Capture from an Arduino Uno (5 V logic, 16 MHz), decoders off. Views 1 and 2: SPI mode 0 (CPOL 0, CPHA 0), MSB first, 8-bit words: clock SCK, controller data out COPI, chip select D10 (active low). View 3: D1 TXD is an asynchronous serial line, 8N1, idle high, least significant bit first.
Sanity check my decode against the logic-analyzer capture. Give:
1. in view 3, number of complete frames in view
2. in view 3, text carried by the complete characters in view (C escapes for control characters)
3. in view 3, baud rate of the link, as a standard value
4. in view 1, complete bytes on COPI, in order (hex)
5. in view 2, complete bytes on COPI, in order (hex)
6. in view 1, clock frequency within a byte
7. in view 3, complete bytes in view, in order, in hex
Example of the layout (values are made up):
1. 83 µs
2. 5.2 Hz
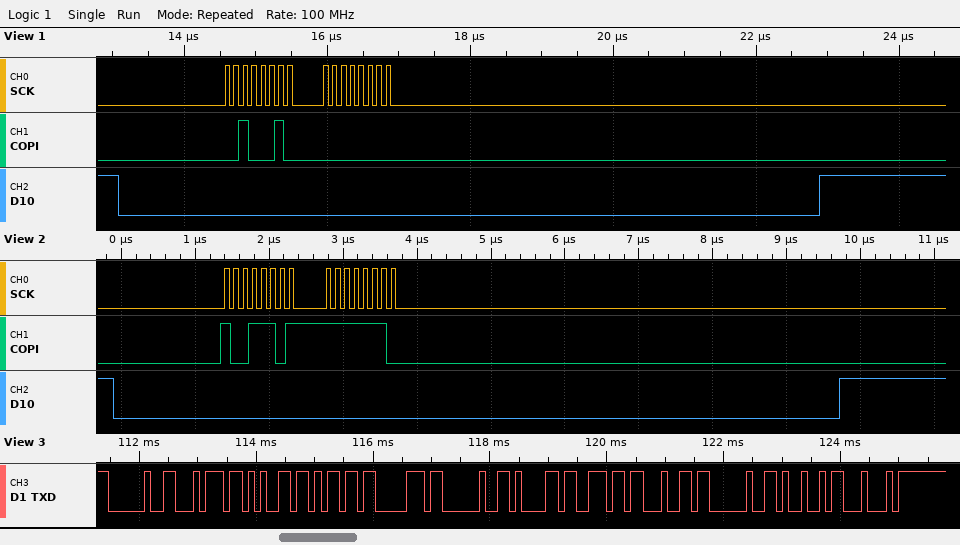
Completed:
1. 12
2. " temp and ID"
3. 9600 baud
4. 22 00
5. 9D FE
6. 8 MHz
7. 20 74 65 6D 70 20 61 6E 64 20 49 44
